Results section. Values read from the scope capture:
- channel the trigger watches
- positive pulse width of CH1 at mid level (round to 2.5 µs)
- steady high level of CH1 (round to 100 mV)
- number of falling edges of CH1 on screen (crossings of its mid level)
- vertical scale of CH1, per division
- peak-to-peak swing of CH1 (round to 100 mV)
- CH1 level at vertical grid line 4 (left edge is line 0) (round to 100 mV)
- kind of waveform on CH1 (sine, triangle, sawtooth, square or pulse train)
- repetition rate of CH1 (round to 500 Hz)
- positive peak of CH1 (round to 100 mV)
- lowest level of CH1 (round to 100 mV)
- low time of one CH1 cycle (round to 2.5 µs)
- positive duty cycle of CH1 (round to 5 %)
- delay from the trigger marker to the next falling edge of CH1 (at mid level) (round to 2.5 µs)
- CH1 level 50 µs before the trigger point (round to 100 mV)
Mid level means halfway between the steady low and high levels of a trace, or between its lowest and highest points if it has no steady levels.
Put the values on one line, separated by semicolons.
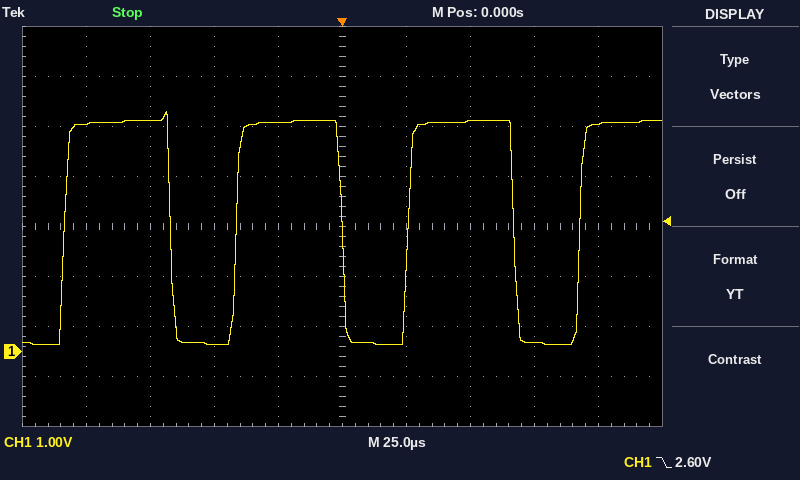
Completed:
CH1; 42.5 µs; 4.6 V; 3; 1 V; 4.7 V; 4.6 V; pulse train; 15.0 kHz; 4.8 V; 100 mV; 25.0 µs; 60 %; 67.5 µs; 100 mV
